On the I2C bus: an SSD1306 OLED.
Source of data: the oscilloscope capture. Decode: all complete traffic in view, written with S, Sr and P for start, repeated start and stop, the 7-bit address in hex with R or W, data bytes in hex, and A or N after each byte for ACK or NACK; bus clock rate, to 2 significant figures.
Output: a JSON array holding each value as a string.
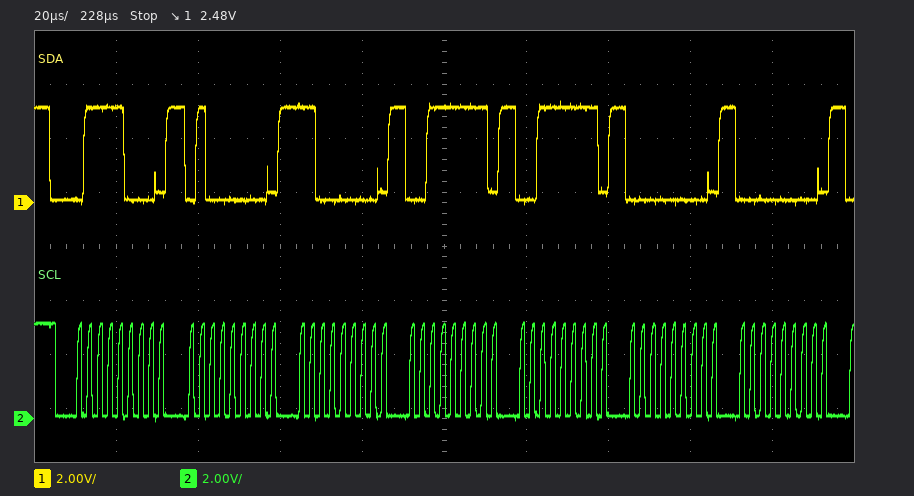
["S 3CW A 40 A C0 A 3F A 3F A 00 A 00 A", "400 kHz"]
